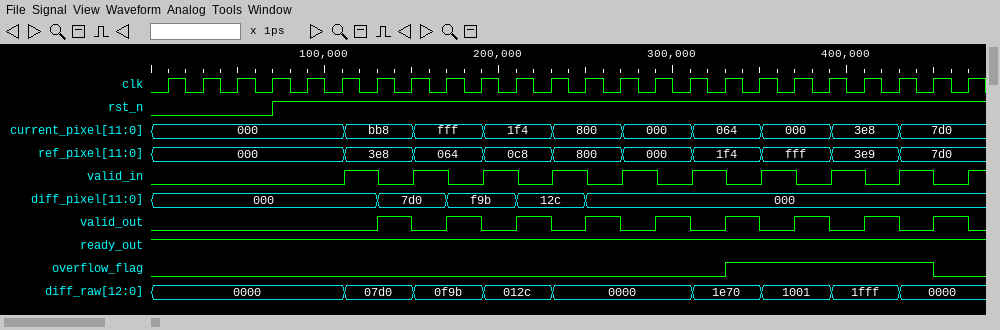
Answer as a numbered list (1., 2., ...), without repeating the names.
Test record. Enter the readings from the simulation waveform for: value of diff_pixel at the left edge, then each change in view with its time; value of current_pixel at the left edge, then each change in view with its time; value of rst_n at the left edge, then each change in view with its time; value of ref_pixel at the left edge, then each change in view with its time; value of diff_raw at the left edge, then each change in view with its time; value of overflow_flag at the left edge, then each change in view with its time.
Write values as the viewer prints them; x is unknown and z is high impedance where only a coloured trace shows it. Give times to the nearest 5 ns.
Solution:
1. 000, 7d0 at 130 ns, f9b at 170 ns, 12c at 210 ns, 000 at 250 ns
2. 000, bb8 at 110 ns, fff at 150 ns, 1f4 at 190 ns, 800 at 230 ns, 000 at 270 ns, 064 at 310 ns, 000 at 350 ns, 3e8 at 390 ns, 7d0 at 430 ns
3. 0, 1 at 70 ns
4. 000, 3e8 at 110 ns, 064 at 150 ns, 0c8 at 190 ns, 800 at 230 ns, 000 at 270 ns, 1f4 at 310 ns, fff at 350 ns, 3e9 at 390 ns, 7d0 at 430 ns
5. 0000, 07d0 at 110 ns, 0f9b at 150 ns, 012c at 190 ns, 0000 at 230 ns, 1e70 at 310 ns, 1001 at 350 ns, 1fff at 390 ns, 0000 at 430 ns
6. 0, 1 at 330 ns, 0 at 450 ns
